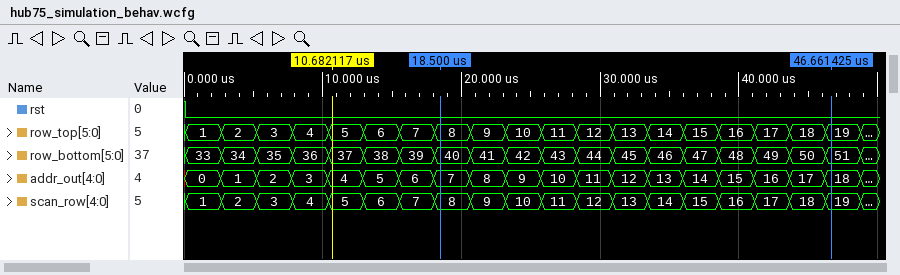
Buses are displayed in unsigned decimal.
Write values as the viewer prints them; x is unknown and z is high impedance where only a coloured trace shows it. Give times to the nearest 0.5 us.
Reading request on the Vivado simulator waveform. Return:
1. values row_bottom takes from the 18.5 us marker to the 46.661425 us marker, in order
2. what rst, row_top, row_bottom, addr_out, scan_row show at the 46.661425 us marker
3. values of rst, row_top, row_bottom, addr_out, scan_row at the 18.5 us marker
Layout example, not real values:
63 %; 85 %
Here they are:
40, 41, 42, 43, 44, 45, 46, 47, 48, 49, 50, 51; rst=0, row_top=19, row_bottom=51, addr_out=18, scan_row=19; rst=0, row_top=8, row_bottom=40, addr_out=7, scan_row=8
